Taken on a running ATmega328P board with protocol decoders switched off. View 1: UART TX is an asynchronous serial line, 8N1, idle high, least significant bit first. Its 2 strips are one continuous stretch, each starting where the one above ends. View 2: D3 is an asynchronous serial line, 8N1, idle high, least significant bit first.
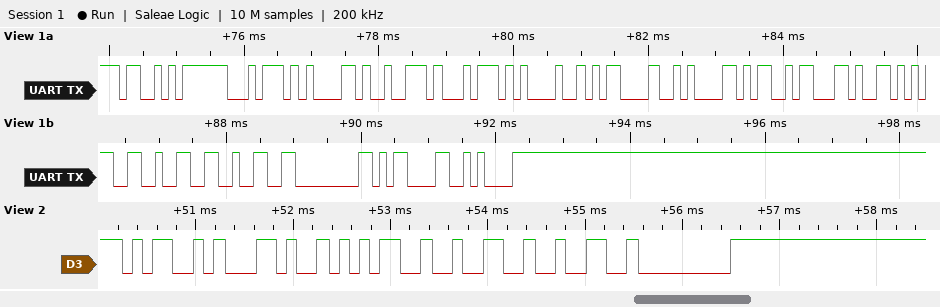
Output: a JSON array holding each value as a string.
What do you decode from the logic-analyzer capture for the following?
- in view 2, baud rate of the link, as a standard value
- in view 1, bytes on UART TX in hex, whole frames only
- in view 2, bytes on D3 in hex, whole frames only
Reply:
["9600 baud", "0x53 0x74 0x61 0x72 0x74 0x21 0x0D 0x0A 0x4D 0x2C 0x35 0x32 0x32 0x00 0x0D 0x0A", "4D 2C 35 32 32 00"]
